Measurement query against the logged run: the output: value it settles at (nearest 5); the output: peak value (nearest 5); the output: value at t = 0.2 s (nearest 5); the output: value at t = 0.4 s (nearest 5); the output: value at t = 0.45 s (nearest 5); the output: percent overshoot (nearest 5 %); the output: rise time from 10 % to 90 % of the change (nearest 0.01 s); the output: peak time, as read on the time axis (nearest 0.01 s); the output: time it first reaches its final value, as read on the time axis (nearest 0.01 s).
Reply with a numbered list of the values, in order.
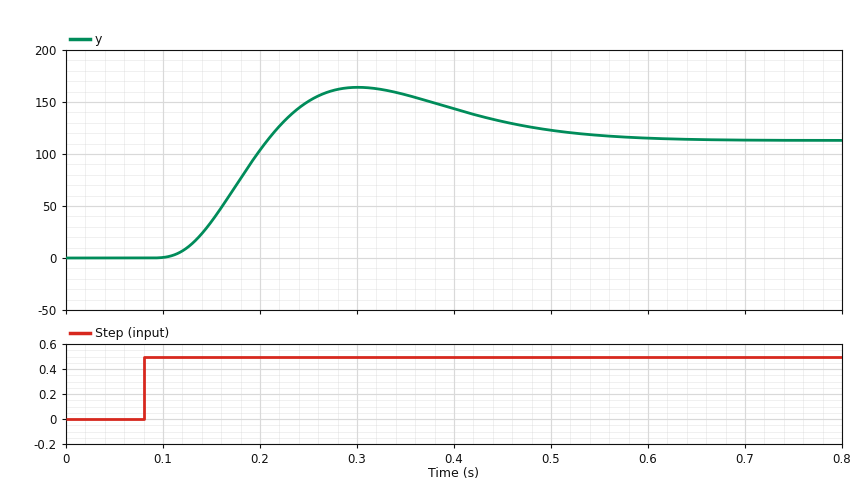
1. 115
2. 165
3. 105
4. 145
5. 130
6. 45 %
7. 0.07 s
8. 0.30 s
9. 0.21 s
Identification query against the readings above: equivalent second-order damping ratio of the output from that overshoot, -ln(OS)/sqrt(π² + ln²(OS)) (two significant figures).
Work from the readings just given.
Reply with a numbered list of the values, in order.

1. 0.25
